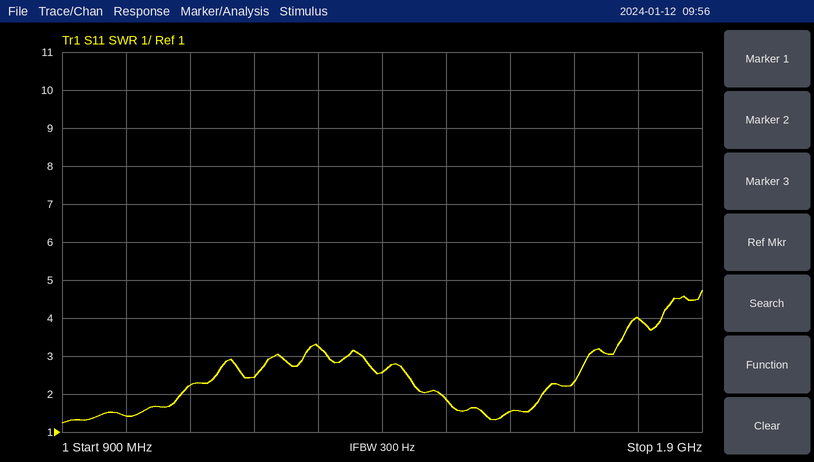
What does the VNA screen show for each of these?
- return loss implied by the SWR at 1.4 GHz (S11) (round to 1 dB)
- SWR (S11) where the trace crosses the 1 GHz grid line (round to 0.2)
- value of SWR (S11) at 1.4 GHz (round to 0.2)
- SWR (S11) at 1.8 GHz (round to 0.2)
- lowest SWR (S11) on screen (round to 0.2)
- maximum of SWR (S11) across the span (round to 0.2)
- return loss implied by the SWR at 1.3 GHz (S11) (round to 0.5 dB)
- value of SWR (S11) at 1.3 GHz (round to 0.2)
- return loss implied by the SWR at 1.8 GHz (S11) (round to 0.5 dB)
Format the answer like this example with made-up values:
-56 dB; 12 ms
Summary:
7 dB; 1.4; 2.6; 4.0; 1.2; 4.8; 5.5 dB; 3.2; 4.5 dB
